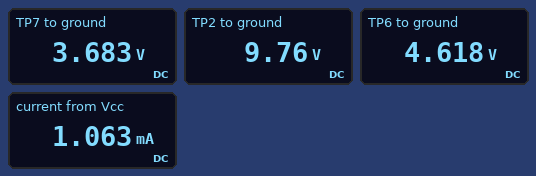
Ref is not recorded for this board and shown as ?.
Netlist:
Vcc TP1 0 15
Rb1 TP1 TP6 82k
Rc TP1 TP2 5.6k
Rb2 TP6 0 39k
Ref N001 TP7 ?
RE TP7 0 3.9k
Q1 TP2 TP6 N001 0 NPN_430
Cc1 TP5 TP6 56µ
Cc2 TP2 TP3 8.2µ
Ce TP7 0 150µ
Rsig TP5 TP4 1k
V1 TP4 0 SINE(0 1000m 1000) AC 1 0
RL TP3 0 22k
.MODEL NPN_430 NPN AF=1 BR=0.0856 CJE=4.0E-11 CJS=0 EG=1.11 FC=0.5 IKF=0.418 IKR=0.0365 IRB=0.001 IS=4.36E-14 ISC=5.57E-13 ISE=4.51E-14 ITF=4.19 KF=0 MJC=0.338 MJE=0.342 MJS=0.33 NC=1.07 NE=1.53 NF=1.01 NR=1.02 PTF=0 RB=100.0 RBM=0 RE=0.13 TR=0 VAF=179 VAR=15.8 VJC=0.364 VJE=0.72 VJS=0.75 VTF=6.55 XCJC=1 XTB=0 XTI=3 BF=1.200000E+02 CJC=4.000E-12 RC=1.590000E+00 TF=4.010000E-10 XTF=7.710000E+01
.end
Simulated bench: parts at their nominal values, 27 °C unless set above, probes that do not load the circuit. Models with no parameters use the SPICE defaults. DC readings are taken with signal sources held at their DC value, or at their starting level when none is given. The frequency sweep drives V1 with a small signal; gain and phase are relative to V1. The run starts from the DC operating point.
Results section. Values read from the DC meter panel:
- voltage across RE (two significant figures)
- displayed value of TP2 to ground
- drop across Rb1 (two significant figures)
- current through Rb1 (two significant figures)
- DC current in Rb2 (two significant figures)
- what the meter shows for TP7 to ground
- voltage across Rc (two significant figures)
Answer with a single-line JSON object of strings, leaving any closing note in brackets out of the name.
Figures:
{"voltage across RE": "3.7 V", "displayed value of TP2 to ground": "9.76 V", "drop across Rb1": "10 V", "current through Rb1": "130 µA", "DC current in Rb2": "120 µA", "what the meter shows for TP7 to ground": "3.683 V", "voltage across Rc": "5.2 V"}
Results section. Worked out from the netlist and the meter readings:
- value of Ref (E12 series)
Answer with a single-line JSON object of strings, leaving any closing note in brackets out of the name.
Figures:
{"value of Ref": "330 Ω"}
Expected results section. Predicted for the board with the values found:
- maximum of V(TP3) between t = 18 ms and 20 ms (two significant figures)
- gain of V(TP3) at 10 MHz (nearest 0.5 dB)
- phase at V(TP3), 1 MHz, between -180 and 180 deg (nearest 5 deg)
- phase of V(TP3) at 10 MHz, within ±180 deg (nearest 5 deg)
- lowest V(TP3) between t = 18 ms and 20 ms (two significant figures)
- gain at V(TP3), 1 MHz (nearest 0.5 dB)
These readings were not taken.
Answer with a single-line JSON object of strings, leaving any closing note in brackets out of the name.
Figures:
{"maximum of V(TP3) between t = 18 ms and 20 ms": "4.2 V", "gain of V(TP3) at 10 MHz": "13.5 dB", "phase at V(TP3), 1 MHz, between -180 and 180 deg": "165 deg", "phase of V(TP3) at 10 MHz, within ±180 deg": "105 deg", "lowest V(TP3) between t = 18 ms and 20 ms": "-5.1 V", "gain at V(TP3), 1 MHz": "21.0 dB"}
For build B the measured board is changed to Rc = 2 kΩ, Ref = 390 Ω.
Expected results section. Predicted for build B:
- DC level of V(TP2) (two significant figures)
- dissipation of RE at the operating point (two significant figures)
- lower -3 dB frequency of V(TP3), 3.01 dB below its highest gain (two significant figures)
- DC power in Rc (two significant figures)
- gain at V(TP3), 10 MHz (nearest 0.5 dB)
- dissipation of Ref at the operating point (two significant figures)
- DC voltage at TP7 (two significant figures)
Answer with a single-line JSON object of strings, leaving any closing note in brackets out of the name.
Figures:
{"DC level of V(TP2)": "13 V", "dissipation of RE at the operating point": "3.4 mW", "lower -3 dB frequency of V(TP3), 3.01 dB below its highest gain": "3.0 Hz", "DC power in Rc": "1.7 mW", "gain at V(TP3), 10 MHz": "9.0 dB", "dissipation of Ref at the operating point": "340 µW", "DC voltage at TP7": "3.6 V"}
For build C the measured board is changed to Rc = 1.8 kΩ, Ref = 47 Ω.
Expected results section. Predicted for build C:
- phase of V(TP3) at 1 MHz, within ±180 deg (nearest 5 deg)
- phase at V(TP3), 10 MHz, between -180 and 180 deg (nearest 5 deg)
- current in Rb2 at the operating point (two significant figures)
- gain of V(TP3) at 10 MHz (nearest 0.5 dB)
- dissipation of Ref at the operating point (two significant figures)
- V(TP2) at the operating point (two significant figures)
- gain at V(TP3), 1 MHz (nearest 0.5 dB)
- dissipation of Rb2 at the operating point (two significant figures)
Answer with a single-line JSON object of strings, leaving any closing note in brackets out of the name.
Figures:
{"phase of V(TP3) at 1 MHz, within ±180 deg": "160 deg", "phase at V(TP3), 10 MHz, between -180 and 180 deg": "100 deg", "current in Rb2 at the operating point": "120 µA", "gain of V(TP3) at 10 MHz": "14.0 dB", "dissipation of Ref at the operating point": "48 µW", "V(TP2) at the operating point": "13 V", "gain at V(TP3), 1 MHz": "25.0 dB", "dissipation of Rb2 at the operating point": "540 µW"}
